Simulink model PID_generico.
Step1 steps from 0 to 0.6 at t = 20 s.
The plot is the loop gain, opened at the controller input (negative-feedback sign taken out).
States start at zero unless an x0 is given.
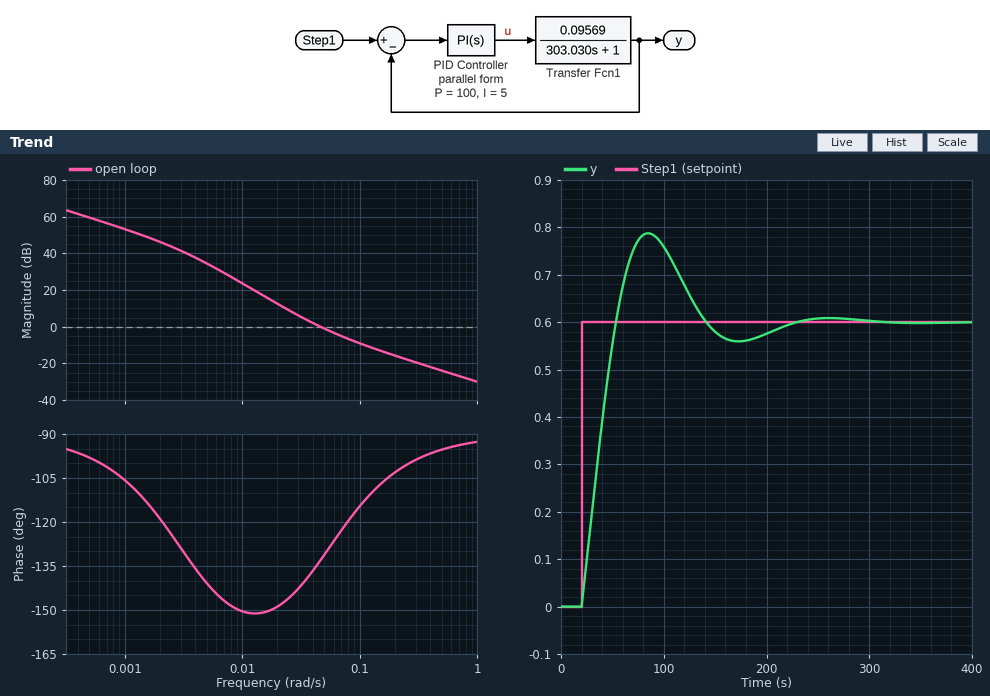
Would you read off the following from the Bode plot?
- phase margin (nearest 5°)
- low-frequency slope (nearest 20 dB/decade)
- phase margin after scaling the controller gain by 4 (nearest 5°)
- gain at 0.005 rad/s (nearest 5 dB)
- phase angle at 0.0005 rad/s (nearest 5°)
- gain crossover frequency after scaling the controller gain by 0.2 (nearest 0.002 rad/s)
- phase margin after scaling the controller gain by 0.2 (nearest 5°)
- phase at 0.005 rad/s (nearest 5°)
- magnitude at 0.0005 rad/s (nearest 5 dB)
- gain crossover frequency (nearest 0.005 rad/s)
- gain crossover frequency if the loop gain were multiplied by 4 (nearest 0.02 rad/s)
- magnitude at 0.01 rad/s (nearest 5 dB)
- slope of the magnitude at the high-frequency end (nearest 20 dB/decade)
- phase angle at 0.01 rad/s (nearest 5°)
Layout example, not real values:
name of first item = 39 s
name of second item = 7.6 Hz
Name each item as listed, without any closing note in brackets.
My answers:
phase margin = 45°
low-frequency slope = -20 dB/decade
phase margin after scaling the controller gain by 4 = 70°
gain at 0.005 rad/s = 35 dB
phase angle at 0.0005 rad/s = -100°
gain crossover frequency after scaling the controller gain by 0.2 = 0.018 rad/s
phase margin after scaling the controller gain by 0.2 = 30°
phase at 0.005 rad/s = -140°
magnitude at 0.0005 rad/s = 60 dB
gain crossover frequency = 0.045 rad/s
gain crossover frequency if the loop gain were multiplied by 4 = 0.14 rad/s
magnitude at 0.01 rad/s = 25 dB
slope of the magnitude at the high-frequency end = -20 dB/decade
phase angle at 0.01 rad/s = -150°
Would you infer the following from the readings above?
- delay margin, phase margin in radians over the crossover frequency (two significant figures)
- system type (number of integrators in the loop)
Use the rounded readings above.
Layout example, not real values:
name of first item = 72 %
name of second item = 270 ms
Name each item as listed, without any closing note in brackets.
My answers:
delay margin, phase margin in radians over the crossover frequency = 17 s
system type = 1
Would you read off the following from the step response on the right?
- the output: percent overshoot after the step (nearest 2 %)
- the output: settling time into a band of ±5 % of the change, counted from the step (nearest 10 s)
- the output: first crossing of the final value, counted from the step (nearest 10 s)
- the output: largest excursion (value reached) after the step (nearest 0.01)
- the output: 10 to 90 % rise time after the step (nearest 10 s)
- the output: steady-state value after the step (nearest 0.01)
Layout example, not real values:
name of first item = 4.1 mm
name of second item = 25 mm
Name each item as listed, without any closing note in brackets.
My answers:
the output: percent overshoot after the step = 32 %
the output: settling time into a band of ±5 % of the change, counted from the step = 170 s
the output: first crossing of the final value, counted from the step = 30 s
the output: largest excursion (value reached) after the step = 0.79
the output: 10 to 90 % rise time after the step = 30 s
the output: steady-state value after the step = 0.60
